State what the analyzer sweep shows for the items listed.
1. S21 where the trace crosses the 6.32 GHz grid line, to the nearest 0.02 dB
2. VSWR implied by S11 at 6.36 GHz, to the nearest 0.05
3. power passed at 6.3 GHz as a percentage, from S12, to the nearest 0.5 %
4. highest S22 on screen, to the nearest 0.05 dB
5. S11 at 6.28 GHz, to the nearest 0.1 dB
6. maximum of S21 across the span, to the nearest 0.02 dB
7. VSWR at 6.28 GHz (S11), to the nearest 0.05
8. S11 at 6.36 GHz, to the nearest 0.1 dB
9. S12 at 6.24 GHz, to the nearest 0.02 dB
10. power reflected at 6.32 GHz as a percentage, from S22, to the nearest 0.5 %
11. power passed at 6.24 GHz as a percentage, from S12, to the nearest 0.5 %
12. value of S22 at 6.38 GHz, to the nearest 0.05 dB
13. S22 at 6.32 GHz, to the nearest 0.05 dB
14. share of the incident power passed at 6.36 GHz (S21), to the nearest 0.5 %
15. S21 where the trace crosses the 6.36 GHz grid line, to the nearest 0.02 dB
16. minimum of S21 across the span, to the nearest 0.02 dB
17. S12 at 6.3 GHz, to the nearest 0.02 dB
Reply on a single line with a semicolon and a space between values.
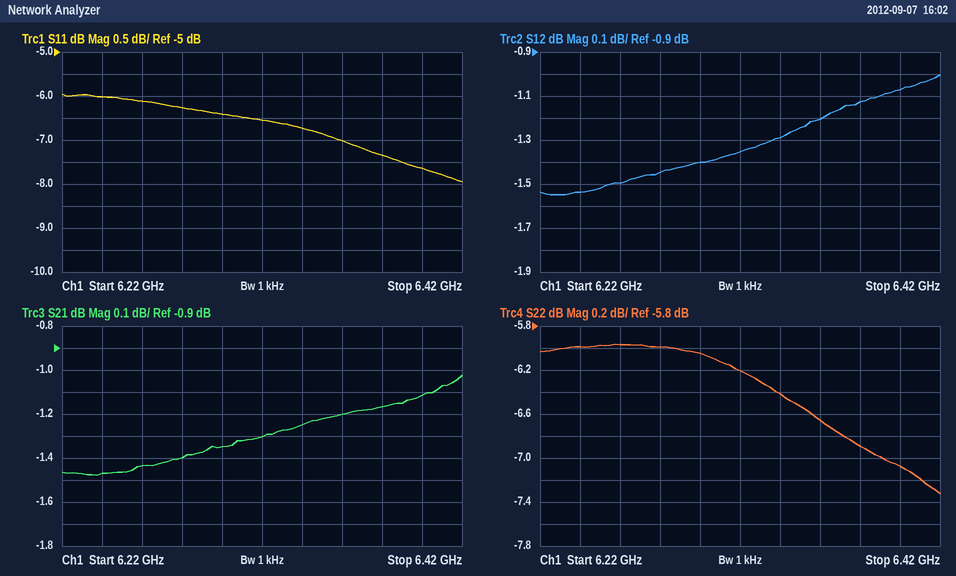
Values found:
-1.30 dB; 2.60; 72.5 %; -5.95 dB; -6.3 dB; -1.02 dB; 2.90; -7.0 dB; -1.54 dB; 24.0 %; 70.0 %; -6.90 dB; -6.20 dB; 76.0 %; -1.20 dB; -1.48 dB; -1.40 dB
